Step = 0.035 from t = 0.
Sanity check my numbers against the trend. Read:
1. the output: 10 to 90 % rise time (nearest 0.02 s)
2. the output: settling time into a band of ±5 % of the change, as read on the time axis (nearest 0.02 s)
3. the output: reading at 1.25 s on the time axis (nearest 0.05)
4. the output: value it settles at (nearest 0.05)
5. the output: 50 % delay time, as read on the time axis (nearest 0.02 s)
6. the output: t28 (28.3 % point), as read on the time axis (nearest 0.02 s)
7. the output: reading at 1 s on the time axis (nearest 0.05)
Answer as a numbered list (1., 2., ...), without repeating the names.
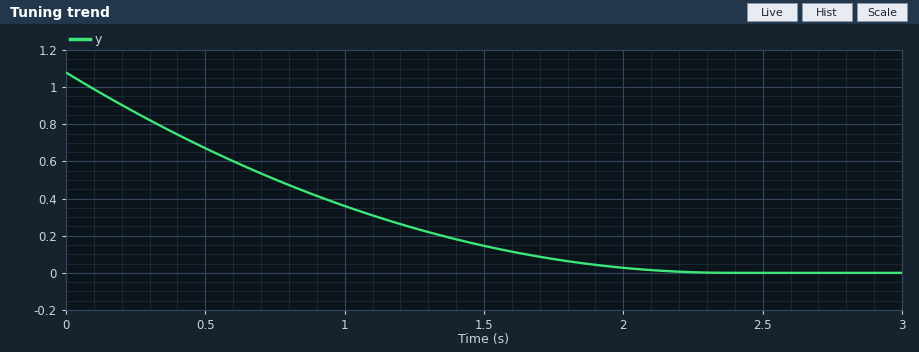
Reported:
1. 1.50 s
2. 1.84 s
3. 0.25
4. 0.00
5. 0.70 s
6. 0.36 s
7. 0.35
